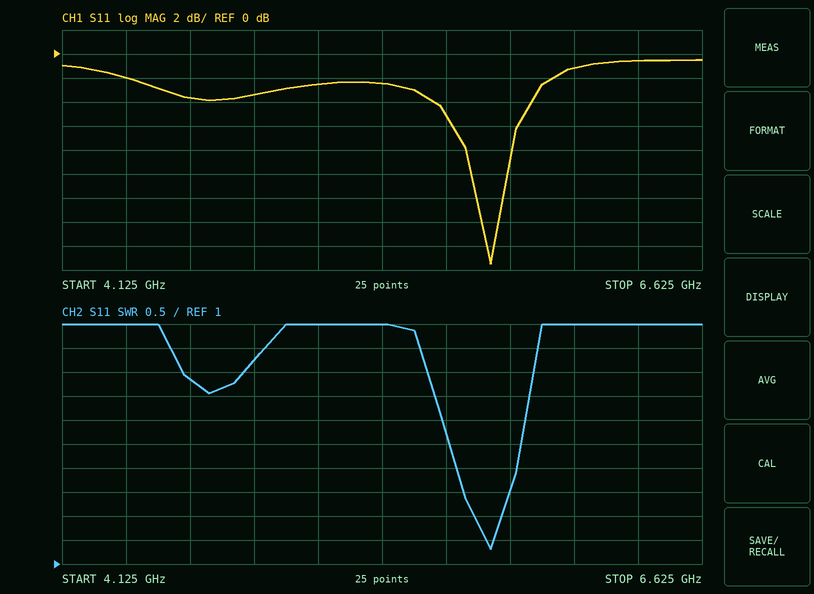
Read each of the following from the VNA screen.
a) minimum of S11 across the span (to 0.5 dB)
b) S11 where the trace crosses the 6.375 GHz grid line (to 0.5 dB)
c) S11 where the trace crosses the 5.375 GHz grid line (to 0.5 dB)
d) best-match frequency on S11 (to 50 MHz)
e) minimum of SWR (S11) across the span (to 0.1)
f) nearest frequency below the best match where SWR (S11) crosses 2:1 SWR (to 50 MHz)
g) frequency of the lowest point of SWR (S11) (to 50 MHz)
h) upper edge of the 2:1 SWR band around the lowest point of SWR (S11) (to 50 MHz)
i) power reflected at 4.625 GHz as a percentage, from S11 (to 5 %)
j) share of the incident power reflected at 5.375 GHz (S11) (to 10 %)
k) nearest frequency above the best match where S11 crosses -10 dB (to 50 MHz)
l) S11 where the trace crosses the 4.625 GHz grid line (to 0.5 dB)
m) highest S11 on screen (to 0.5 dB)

-17.5 dB
-0.5 dB
-2.5 dB
5.80 GHz
1.3
5.75 GHz
5.80 GHz
5.85 GHz
45 %
60 %
5.85 GHz
-3.5 dB
-0.5 dB
